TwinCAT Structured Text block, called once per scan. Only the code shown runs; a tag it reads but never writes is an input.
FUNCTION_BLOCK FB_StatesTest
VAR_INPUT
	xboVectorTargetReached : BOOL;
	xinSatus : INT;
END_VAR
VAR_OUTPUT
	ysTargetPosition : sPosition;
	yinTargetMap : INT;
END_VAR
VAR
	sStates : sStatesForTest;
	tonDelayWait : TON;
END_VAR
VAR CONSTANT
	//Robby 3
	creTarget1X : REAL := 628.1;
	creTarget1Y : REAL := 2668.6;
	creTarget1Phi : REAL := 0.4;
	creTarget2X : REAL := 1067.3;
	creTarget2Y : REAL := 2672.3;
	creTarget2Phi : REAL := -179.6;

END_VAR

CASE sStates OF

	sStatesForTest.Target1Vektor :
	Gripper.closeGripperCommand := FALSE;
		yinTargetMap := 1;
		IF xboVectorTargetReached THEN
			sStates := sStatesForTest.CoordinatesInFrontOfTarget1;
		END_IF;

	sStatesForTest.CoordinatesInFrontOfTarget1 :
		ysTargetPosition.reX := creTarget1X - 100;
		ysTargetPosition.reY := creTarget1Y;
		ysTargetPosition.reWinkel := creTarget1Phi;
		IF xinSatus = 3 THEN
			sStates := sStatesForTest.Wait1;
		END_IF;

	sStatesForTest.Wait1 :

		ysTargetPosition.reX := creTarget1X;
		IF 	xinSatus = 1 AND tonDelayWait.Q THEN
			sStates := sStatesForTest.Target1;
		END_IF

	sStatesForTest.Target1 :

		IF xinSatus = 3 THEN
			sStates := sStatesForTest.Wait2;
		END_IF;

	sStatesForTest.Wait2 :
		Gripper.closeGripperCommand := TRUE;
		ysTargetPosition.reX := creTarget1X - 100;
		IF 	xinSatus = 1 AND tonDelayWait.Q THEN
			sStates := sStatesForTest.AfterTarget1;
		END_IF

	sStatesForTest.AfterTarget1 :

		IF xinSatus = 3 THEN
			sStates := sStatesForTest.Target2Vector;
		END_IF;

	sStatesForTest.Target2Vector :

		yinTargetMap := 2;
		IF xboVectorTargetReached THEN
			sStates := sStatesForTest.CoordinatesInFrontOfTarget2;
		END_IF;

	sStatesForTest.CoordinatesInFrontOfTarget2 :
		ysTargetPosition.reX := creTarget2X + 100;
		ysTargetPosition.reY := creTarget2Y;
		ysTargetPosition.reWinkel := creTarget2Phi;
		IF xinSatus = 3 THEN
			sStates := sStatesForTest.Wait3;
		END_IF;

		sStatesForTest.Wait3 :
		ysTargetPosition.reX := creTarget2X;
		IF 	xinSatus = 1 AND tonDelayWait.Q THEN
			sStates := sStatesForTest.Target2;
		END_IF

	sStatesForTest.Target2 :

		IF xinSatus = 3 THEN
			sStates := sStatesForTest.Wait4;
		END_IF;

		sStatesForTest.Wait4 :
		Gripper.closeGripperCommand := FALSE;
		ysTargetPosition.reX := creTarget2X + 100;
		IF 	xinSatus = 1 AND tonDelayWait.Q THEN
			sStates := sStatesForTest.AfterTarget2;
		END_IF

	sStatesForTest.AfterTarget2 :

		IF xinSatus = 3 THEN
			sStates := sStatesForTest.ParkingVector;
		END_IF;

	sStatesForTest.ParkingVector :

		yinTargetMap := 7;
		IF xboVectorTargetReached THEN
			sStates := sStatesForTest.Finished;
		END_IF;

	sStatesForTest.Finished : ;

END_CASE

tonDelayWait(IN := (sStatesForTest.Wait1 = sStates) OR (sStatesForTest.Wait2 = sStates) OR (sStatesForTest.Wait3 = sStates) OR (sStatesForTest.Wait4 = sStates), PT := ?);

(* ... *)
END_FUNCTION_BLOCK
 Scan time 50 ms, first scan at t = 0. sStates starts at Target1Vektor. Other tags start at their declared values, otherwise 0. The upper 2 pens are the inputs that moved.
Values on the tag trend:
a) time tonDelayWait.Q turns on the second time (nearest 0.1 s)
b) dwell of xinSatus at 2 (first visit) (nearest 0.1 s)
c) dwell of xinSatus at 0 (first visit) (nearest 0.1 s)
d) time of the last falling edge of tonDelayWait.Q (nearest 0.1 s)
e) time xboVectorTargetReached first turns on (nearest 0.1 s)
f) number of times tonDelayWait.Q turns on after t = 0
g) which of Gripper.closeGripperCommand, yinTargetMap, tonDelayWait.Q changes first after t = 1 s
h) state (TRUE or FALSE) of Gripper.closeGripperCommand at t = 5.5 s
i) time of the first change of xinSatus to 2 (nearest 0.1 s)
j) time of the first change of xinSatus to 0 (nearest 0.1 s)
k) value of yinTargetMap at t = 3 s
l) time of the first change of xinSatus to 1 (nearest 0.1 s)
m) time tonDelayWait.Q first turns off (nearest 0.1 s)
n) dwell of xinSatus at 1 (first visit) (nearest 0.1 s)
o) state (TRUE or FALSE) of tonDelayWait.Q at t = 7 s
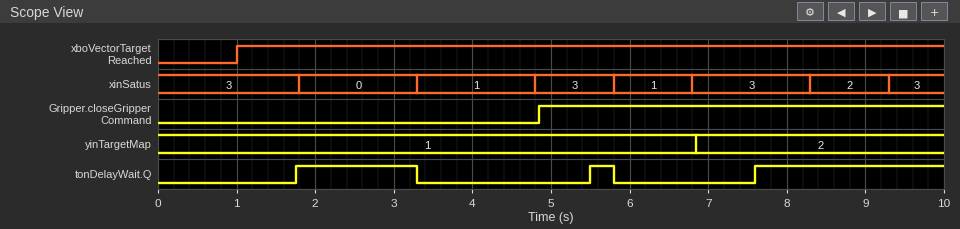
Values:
5.5 s
1.0 s
1.5 s
5.8 s
1.0 s
3
tonDelayWait.Q
TRUE
8.3 s
1.8 s
1
3.3 s
3.3 s
1.5 s
FALSE
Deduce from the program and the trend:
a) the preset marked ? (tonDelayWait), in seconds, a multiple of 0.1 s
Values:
0.7 s
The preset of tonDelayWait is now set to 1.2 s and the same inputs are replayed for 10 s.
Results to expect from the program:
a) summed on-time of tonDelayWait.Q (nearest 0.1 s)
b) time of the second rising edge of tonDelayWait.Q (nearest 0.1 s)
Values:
3.0 s
6.0 s
